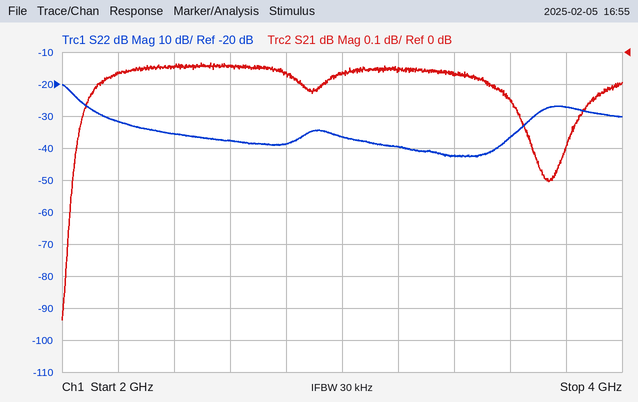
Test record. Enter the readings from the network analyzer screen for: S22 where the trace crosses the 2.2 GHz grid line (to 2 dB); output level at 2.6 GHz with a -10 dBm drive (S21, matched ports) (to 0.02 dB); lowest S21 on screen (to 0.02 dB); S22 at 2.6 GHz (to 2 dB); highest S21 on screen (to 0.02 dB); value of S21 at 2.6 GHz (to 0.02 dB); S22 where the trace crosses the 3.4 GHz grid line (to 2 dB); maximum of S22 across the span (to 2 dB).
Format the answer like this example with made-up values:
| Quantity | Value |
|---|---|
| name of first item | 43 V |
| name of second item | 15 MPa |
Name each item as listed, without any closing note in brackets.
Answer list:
| Quantity | Value |
|---|---|
| S22 where the trace crosses the 2.2 GHz grid line | -32 dB |
| output level at 2.6 GHz with a -10 dBm drive (S21, matched ports) | -10.04 dBm |
| lowest S21 on screen | -0.84 dB |
| S22 at 2.6 GHz | -38 dB |
| highest S21 on screen | -0.04 dB |
| value of S21 at 2.6 GHz | -0.04 dB |
| S22 where the trace crosses the 3.4 GHz grid line | -42 dB |
| maximum of S22 across the span | -20 dB |
